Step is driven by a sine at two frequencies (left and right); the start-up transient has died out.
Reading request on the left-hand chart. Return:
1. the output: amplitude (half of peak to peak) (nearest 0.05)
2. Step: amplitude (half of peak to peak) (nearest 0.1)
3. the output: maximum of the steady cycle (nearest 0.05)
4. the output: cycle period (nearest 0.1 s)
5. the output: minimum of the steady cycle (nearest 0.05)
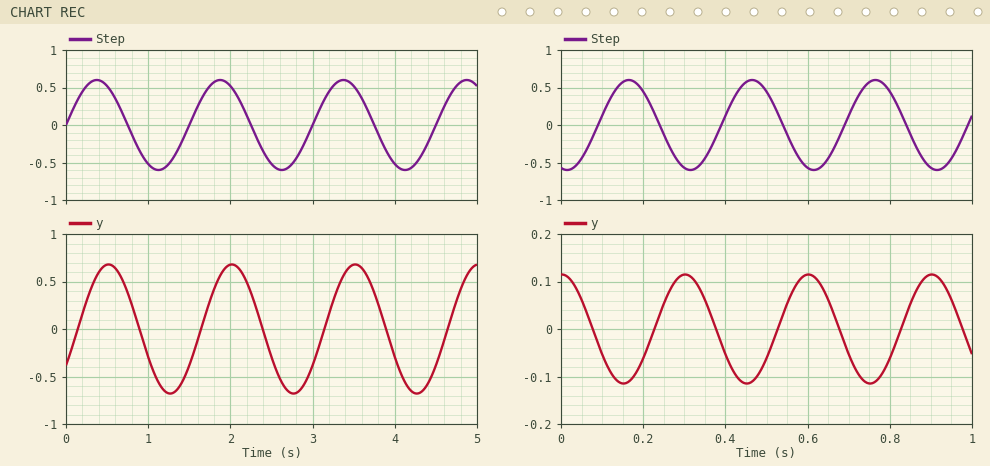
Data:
0.70
0.6
0.70
1.5 s
-0.70
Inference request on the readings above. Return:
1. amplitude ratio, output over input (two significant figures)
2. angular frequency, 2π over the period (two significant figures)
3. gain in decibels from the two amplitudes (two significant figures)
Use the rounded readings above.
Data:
1.2
4.2 rad/s
1.3 dB
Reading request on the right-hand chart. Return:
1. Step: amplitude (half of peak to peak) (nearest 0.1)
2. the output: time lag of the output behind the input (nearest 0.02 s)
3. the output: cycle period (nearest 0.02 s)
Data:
0.6
0.14 s
0.30 s
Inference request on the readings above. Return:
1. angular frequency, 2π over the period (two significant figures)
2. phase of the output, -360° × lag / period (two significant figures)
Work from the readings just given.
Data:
21 rad/s
-170°
